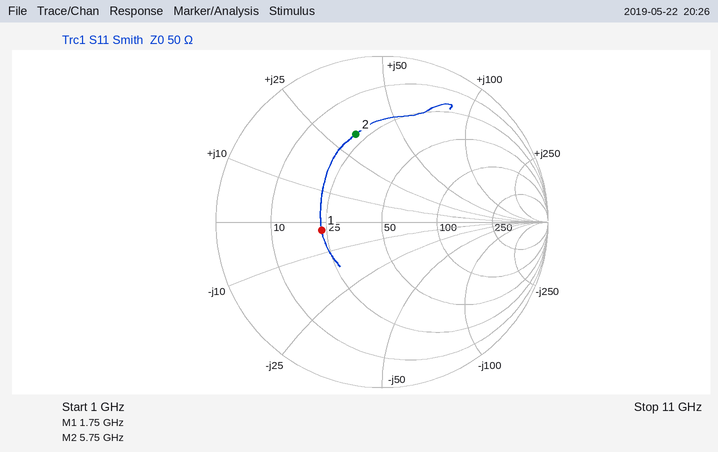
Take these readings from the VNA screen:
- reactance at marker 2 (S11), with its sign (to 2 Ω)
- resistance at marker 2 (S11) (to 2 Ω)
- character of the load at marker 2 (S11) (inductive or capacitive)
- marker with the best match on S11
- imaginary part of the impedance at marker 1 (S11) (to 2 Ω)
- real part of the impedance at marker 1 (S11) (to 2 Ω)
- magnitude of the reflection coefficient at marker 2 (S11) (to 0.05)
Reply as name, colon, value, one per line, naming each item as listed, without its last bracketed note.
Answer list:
reactance at marker 2 (S11), with its sign: +32 Ω
resistance at marker 2 (S11): 22 Ω
character of the load at marker 2 (S11): inductive
marker with the best match on S11: marker 1
imaginary part of the impedance at marker 1 (S11): -2 Ω
real part of the impedance at marker 1 (S11): 24 Ω
magnitude of the reflection coefficient at marker 2 (S11): 0.55
